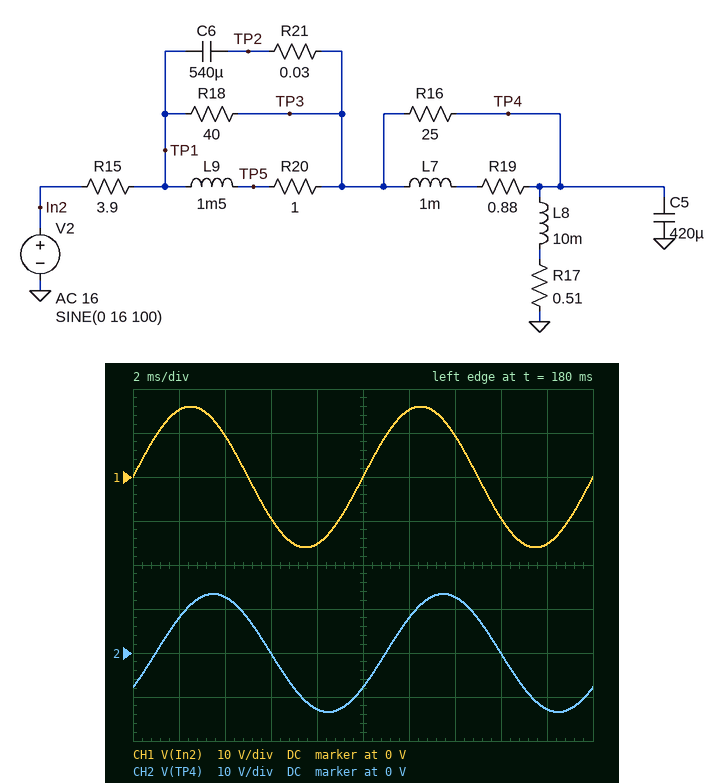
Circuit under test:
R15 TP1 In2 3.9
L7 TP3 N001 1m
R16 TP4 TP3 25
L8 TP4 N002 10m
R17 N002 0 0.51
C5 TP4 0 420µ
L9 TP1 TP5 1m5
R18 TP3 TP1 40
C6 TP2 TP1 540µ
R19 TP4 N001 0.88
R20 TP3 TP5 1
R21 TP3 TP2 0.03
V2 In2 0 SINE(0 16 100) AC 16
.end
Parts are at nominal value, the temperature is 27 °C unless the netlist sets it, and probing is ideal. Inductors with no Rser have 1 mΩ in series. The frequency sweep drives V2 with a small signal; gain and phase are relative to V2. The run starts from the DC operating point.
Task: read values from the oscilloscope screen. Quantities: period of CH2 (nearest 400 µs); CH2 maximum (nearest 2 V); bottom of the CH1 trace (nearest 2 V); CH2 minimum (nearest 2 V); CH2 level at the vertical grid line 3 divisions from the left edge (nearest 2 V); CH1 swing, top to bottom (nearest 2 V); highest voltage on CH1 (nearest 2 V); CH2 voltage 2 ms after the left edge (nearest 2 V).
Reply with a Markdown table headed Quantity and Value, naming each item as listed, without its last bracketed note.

| Quantity | Value |
|---|---|
| period of CH2 | 10.0 ms |
| CH2 maximum | 14 V |
| bottom of the CH1 trace | -16 V |
| CH2 minimum | -14 V |
| CH2 level at the vertical grid line 3 divisions from the left edge | 0 V |
| CH1 swing, top to bottom | 32 V |
| highest voltage on CH1 | 16 V |
| CH2 voltage 2 ms after the left edge | 8 V |
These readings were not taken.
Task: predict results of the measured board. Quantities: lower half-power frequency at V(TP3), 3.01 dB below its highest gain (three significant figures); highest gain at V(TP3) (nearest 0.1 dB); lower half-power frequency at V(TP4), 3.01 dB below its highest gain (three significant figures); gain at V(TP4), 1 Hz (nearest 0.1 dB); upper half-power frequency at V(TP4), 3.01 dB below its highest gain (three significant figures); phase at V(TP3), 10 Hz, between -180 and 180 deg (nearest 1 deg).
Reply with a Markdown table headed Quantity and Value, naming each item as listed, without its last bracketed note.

| Quantity | Value |
|---|---|
| lower half-power frequency at V(TP3), 3.01 dB below its highest gain | 50.3 Hz |
| highest gain at V(TP3) | -0.8 dB |
| lower half-power frequency at V(TP4), 3.01 dB below its highest gain | 54.7 Hz |
| gain at V(TP4), 1 Hz | -21.7 dB |
| upper half-power frequency at V(TP4), 3.01 dB below its highest gain | 121 Hz |
| phase at V(TP3), 10 Hz, between -180 and 180 deg | 20 deg |
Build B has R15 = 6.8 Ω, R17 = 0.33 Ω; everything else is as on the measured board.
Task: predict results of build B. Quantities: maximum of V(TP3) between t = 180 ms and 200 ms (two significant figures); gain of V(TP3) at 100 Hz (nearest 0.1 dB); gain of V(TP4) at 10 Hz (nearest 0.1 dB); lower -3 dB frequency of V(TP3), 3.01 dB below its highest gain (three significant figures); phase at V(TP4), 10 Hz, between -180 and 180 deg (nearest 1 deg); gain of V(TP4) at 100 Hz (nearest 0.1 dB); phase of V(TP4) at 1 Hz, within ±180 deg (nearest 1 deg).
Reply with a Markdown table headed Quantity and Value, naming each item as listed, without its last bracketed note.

| Quantity | Value |
|---|---|
| maximum of V(TP3) between t = 180 ms and 200 ms | 11 V |
| gain of V(TP3) at 100 Hz | -3.3 dB |
| gain of V(TP4) at 10 Hz | -21.9 dB |
| lower -3 dB frequency of V(TP3), 3.01 dB below its highest gain | 57.8 Hz |
| phase at V(TP4), 10 Hz, between -180 and 180 deg | 57 deg |
| gain of V(TP4) at 100 Hz | -2.8 dB |
| phase of V(TP4) at 1 Hz, within ±180 deg | 10 deg |
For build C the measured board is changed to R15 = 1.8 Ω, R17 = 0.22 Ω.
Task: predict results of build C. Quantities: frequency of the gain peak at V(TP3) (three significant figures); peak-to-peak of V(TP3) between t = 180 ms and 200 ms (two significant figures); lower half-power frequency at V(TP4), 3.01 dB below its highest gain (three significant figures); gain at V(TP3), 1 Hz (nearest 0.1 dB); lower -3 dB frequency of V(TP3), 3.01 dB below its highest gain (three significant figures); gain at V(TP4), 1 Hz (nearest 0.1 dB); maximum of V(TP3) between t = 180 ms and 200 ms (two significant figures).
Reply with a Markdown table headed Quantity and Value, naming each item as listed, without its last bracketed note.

| Quantity | Value |
|---|---|
| frequency of the gain peak at V(TP3) | 84.0 Hz |
| peak-to-peak of V(TP3) between t = 180 ms and 200 ms | 30 V |
| lower half-power frequency at V(TP4), 3.01 dB below its highest gain | 48.0 Hz |
| gain at V(TP3), 1 Hz | -11.1 dB |
| lower -3 dB frequency of V(TP3), 3.01 dB below its highest gain | 41.0 Hz |
| gain at V(TP4), 1 Hz | -24.5 dB |
| maximum of V(TP3) between t = 180 ms and 200 ms | 15 V |
